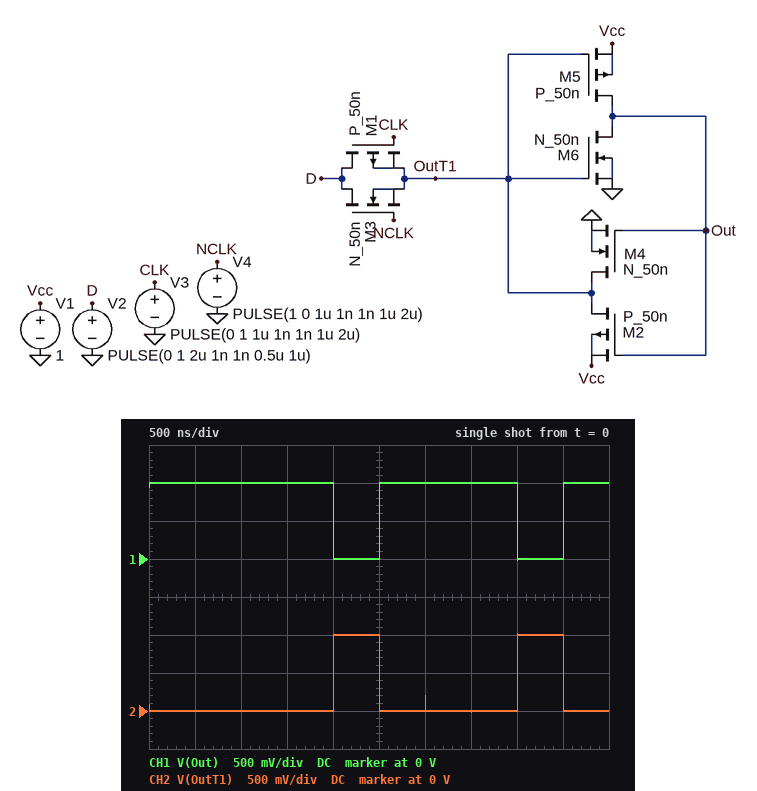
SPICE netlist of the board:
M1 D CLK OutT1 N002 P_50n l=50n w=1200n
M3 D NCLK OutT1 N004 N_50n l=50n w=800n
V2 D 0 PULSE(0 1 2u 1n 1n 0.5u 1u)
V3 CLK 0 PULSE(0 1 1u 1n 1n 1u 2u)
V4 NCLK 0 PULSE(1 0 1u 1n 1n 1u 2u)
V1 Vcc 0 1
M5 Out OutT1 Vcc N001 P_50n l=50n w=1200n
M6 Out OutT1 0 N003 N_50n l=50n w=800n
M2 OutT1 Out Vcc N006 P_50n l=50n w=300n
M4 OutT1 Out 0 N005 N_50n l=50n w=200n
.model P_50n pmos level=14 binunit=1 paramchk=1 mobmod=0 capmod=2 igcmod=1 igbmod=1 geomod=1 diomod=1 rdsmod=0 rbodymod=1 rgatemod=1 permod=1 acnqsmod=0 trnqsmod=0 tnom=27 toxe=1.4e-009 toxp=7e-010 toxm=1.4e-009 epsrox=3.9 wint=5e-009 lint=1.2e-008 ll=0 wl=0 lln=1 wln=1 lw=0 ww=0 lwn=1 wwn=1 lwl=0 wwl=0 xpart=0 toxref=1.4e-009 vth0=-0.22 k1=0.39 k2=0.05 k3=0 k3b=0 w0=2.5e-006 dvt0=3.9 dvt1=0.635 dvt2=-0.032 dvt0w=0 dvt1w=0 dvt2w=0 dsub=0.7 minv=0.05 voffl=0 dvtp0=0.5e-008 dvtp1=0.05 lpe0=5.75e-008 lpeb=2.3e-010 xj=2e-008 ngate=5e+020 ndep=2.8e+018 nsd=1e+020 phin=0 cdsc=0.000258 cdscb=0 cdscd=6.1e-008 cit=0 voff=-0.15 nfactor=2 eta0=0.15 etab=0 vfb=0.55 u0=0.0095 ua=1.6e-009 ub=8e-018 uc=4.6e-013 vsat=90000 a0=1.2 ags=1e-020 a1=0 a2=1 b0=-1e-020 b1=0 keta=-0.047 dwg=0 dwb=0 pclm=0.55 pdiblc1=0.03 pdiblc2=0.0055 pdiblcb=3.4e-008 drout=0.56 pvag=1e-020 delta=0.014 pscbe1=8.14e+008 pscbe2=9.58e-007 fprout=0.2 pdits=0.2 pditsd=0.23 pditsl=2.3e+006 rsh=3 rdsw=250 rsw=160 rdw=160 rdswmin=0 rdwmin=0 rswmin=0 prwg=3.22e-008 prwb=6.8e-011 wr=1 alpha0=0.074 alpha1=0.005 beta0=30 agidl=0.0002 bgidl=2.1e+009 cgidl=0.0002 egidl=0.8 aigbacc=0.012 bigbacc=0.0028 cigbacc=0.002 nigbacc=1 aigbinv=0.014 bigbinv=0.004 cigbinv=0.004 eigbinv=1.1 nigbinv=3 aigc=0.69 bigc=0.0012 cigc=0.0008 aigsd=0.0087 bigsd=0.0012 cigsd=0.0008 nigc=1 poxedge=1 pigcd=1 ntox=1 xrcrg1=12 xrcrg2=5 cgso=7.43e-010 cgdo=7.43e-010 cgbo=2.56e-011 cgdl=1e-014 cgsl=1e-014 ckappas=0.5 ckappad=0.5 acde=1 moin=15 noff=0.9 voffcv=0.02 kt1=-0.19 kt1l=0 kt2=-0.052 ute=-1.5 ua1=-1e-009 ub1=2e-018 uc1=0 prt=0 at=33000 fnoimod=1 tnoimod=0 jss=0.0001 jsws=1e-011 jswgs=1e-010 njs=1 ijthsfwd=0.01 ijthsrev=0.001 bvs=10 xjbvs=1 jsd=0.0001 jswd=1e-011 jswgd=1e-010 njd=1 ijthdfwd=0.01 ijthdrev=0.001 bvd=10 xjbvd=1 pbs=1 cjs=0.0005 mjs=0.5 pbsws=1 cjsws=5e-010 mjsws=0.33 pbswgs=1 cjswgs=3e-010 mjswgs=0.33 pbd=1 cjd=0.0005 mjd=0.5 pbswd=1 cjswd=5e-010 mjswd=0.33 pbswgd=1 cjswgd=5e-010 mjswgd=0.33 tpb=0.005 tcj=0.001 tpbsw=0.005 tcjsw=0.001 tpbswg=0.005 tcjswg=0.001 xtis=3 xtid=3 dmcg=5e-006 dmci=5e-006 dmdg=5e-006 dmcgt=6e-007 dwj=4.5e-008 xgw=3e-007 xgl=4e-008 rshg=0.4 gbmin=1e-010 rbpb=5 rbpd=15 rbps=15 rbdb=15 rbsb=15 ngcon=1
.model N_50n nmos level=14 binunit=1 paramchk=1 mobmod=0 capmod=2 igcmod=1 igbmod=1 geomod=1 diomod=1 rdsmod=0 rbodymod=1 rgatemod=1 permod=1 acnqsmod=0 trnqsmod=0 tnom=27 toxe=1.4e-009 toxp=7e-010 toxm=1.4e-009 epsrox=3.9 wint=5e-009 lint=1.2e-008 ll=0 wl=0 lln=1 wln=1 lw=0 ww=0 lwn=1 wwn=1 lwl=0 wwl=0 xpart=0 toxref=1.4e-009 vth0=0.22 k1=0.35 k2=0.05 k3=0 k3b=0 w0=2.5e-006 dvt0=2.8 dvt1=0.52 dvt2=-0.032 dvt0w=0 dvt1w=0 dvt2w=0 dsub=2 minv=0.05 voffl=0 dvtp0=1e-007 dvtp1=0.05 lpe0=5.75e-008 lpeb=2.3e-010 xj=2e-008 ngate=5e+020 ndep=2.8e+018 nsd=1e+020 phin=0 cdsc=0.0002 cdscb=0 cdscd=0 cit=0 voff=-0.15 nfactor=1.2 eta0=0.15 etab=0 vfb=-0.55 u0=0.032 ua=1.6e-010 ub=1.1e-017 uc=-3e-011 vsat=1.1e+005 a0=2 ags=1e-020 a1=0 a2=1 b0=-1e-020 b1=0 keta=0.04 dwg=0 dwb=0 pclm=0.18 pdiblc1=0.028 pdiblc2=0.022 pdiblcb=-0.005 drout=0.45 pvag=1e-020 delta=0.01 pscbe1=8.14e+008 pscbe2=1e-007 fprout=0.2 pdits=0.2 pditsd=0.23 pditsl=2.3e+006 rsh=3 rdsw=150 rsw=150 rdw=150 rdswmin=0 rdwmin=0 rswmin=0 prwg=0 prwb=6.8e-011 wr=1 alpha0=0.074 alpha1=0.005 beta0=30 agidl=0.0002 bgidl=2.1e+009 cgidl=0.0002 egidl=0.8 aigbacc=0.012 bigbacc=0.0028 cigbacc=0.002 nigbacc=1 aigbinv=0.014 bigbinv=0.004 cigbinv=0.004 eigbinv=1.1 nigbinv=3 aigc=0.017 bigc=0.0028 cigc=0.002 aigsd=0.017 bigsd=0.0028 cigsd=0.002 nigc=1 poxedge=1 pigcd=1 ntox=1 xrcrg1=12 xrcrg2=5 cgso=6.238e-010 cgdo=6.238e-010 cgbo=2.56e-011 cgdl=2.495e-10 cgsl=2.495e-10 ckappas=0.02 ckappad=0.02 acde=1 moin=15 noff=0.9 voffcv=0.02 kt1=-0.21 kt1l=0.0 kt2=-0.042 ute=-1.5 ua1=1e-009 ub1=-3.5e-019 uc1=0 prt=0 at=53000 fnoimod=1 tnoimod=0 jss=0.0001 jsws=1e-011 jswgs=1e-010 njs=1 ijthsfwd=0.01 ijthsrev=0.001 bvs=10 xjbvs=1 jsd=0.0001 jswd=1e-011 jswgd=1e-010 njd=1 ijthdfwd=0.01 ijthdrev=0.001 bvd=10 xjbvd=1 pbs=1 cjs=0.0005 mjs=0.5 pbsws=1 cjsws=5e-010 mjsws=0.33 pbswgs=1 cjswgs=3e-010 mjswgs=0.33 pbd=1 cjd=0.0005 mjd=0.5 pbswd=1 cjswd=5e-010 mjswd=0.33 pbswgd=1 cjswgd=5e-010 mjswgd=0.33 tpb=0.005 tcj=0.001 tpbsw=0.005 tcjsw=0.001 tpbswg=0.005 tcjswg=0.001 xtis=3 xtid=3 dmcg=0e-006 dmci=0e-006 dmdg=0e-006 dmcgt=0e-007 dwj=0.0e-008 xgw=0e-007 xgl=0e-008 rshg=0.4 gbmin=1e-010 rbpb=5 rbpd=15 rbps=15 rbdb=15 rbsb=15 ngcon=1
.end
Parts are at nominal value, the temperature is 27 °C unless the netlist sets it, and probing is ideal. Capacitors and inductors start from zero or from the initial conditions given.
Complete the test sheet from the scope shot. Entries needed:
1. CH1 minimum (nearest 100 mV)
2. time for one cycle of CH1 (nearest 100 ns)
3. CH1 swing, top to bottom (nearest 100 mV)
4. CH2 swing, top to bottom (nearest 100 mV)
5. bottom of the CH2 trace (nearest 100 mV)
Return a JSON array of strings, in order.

["0 V", "2.0 µs", "1.0 V", "1.0 V", "0 V"]
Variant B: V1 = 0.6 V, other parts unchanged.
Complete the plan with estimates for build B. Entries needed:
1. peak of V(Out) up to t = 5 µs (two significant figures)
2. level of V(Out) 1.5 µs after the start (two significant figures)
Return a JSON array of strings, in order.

["610 mV", "600 mV"]
